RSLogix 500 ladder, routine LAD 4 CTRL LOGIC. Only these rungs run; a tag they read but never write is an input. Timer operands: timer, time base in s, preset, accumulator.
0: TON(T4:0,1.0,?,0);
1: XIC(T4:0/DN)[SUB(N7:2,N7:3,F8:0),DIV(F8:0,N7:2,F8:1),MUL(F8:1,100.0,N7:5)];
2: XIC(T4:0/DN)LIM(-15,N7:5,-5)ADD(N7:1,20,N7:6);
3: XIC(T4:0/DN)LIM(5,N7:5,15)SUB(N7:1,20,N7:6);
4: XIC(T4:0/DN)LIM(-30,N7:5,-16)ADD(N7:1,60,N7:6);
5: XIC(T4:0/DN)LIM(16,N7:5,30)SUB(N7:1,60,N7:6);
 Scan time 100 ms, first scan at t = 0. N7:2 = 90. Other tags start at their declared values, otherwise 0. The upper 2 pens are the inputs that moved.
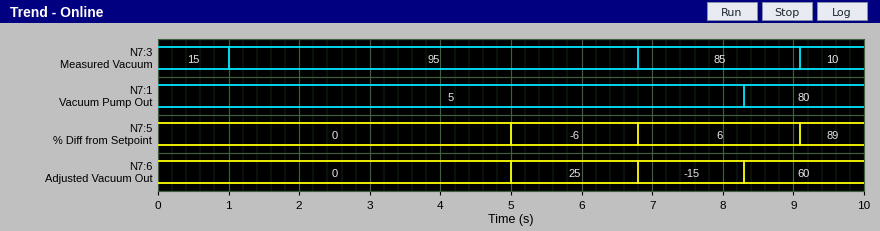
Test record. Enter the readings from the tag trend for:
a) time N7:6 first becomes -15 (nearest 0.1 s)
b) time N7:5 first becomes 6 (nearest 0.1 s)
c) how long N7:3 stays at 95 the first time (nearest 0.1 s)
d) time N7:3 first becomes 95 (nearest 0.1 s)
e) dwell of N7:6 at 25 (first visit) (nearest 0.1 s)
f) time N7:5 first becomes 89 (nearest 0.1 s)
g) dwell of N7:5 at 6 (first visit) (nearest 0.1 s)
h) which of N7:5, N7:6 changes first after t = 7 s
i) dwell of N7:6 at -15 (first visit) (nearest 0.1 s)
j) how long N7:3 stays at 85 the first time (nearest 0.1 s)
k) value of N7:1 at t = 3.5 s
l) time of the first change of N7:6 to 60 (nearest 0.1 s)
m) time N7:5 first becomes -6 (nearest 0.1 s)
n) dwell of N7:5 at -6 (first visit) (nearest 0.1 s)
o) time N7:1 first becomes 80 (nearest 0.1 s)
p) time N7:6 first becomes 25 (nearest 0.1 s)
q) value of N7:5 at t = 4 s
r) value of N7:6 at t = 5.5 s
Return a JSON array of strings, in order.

["6.8 s", "6.8 s", "5.8 s", "1.0 s", "1.8 s", "9.1 s", "2.3 s", "N7:6", "1.5 s", "2.3 s", "5", "8.3 s", "5.0 s", "1.8 s", "8.3 s", "5.0 s", "0", "25"]
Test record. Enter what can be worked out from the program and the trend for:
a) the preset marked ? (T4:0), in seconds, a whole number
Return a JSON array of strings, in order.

["5 s"]
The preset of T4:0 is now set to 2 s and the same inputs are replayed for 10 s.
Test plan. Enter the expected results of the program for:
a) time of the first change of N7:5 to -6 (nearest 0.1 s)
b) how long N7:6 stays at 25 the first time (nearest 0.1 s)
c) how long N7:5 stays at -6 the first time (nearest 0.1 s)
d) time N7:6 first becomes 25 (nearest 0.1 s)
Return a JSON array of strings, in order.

["2.0 s", "4.8 s", "4.8 s", "2.0 s"]
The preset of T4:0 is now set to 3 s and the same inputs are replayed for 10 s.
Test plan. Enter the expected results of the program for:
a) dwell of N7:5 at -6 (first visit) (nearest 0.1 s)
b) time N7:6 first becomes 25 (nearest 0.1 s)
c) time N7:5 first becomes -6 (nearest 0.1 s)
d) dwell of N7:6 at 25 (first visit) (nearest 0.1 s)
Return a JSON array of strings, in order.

["3.8 s", "3.0 s", "3.0 s", "3.8 s"]
